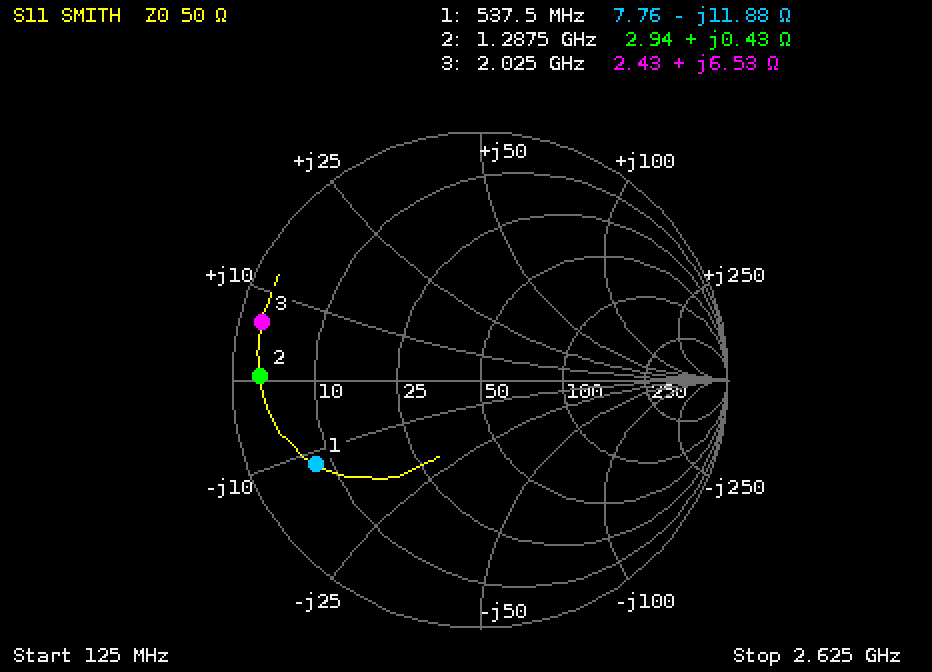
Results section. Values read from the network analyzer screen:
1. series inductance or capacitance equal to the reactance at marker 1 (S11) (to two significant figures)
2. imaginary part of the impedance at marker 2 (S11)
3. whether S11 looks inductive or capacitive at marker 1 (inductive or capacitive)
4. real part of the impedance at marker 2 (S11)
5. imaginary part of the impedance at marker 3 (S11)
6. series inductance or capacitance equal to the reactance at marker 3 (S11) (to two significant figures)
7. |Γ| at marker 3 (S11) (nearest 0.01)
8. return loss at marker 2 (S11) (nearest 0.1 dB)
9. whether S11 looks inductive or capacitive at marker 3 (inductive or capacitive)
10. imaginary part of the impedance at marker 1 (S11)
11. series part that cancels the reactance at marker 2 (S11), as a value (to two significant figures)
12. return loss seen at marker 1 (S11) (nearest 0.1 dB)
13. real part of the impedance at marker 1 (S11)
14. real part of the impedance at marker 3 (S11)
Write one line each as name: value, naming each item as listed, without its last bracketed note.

series inductance or capacitance equal to the reactance at marker 1 (S11): 25 pF
imaginary part of the impedance at marker 2: +0.43 Ω
whether S11 looks inductive or capacitive at marker 1: capacitive
real part of the impedance at marker 2: 2.94 Ω
imaginary part of the impedance at marker 3: +6.53 Ω
series inductance or capacitance equal to the reactance at marker 3 (S11): 510 pH
|Γ| at marker 3 (S11): 0.91
return loss at marker 2 (S11): 1.0 dB
whether S11 looks inductive or capacitive at marker 3: inductive
imaginary part of the impedance at marker 1: -11.88 Ω
series part that cancels the reactance at marker 2 (S11), as a value: 290 pF
return loss seen at marker 1 (S11): 2.6 dB
real part of the impedance at marker 1: 7.76 Ω
real part of the impedance at marker 3: 2.43 Ω
